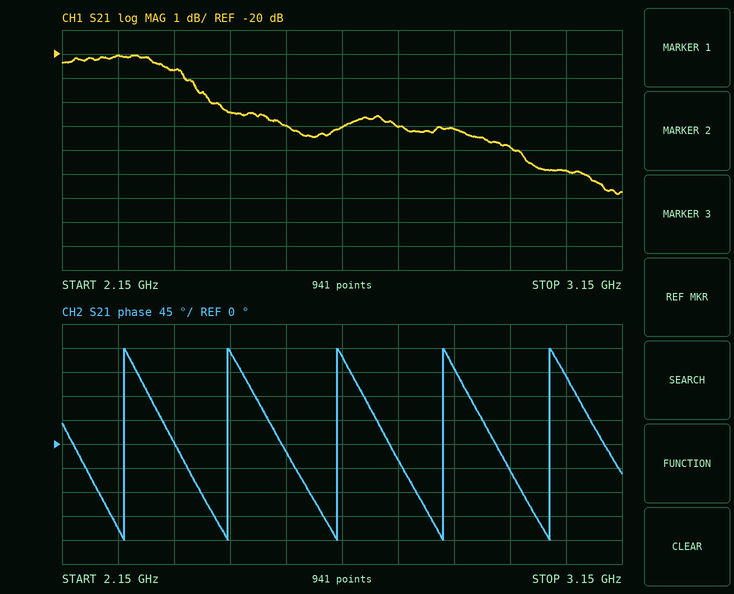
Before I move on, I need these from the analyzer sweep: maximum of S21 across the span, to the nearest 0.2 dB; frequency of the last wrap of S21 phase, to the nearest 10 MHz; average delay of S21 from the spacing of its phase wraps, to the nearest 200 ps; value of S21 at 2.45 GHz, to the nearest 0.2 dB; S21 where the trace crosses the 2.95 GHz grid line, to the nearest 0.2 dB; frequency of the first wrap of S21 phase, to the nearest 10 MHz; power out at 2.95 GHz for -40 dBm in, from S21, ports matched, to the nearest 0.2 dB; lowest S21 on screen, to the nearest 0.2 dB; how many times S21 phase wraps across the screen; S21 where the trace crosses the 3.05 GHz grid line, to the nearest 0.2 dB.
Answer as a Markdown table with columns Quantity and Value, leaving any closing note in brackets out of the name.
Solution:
| Quantity | Value |
|---|---|
| maximum of S21 across the span, to the nearest 0.2 dB | -20.0 dB |
| frequency of the last wrap of S21 phase, to the nearest 10 MHz | 3.02 GHz |
| average delay of S21 from the spacing of its phase wraps, to the nearest 200 ps | 5.2 ns |
| value of S21 at 2.45 GHz, to the nearest 0.2 dB | -22.4 dB |
| S21 where the trace crosses the 2.95 GHz grid line, to the nearest 0.2 dB | -23.8 dB |
| frequency of the first wrap of S21 phase, to the nearest 10 MHz | 2.26 GHz |
| power out at 2.95 GHz for -40 dBm in, from S21, ports matched, to the nearest 0.2 dB | -63.8 dBm |
| lowest S21 on screen, to the nearest 0.2 dB | -25.8 dB |
| how many times S21 phase wraps across the screen | 5 |
| S21 where the trace crosses the 3.05 GHz grid line, to the nearest 0.2 dB | -24.8 dB |
